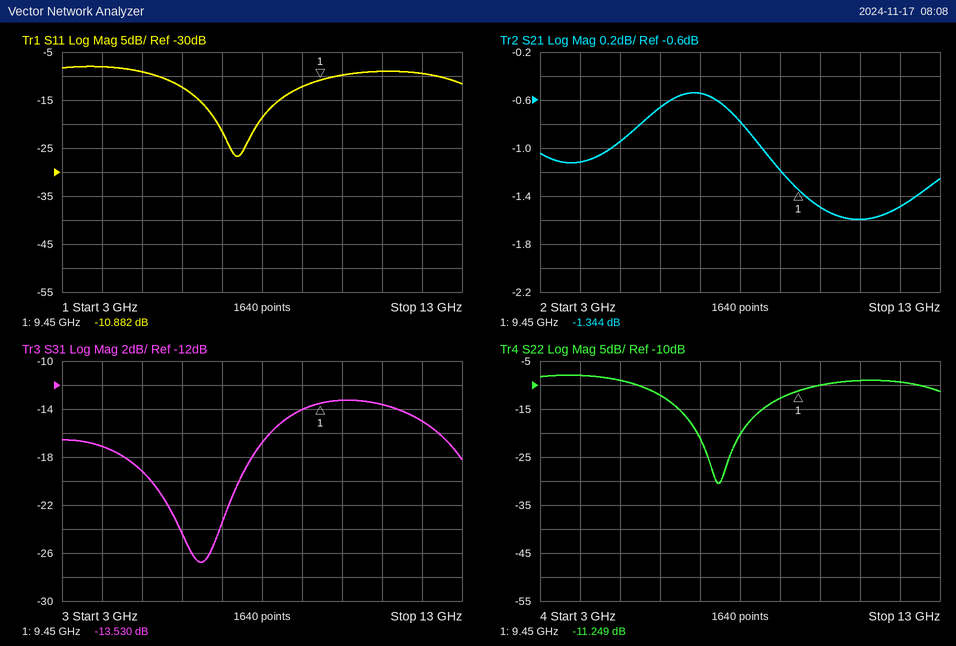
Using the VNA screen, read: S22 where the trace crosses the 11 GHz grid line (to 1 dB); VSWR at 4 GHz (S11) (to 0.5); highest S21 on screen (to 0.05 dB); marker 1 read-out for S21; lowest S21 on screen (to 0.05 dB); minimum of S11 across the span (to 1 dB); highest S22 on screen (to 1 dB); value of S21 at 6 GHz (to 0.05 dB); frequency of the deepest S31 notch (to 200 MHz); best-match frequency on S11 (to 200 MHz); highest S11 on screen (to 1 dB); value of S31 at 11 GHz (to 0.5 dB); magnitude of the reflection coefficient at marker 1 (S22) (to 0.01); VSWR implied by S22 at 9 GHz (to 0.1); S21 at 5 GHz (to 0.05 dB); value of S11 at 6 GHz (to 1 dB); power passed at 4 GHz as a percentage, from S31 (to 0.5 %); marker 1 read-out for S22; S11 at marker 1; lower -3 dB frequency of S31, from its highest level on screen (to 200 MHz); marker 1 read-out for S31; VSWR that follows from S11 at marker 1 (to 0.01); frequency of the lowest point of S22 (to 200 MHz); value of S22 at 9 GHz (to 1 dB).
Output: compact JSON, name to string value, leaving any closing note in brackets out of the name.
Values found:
{"S22 where the trace crosses the 11 GHz grid line": "-9 dB", "VSWR at 4 GHz (S11)": "2.5", "highest S21 on screen": "-0.55 dB", "marker 1 read-out for S21": "-1.344 dB", "lowest S21 on screen": "-1.60 dB", "minimum of S11 across the span": "-27 dB", "highest S22 on screen": "-8 dB", "value of S21 at 6 GHz": "-0.65 dB", "frequency of the deepest S31 notch": "6.4 GHz", "best-match frequency on S11": "7.4 GHz", "highest S11 on screen": "-8 dB", "value of S31 at 11 GHz": "-13.5 dB", "magnitude of the reflection coefficient at marker 1 (S22)": "0.27", "VSWR implied by S22 at 9 GHz": "1.6", "S21 at 5 GHz": "-0.95 dB", "value of S11 at 6 GHz": "-12 dB", "power passed at 4 GHz as a percentage, from S31": "2.0 %", "marker 1 read-out for S22": "-11.249 dB", "S11 at marker 1": "-10.882 dB", "lower -3 dB frequency of S31, from its highest level on screen": "8.2 GHz", "marker 1 read-out for S31": "-13.530 dB", "VSWR that follows from S11 at marker 1": "1.80", "frequency of the lowest point of S22": "7.4 GHz", "value of S22 at 9 GHz": "-13 dB"}
